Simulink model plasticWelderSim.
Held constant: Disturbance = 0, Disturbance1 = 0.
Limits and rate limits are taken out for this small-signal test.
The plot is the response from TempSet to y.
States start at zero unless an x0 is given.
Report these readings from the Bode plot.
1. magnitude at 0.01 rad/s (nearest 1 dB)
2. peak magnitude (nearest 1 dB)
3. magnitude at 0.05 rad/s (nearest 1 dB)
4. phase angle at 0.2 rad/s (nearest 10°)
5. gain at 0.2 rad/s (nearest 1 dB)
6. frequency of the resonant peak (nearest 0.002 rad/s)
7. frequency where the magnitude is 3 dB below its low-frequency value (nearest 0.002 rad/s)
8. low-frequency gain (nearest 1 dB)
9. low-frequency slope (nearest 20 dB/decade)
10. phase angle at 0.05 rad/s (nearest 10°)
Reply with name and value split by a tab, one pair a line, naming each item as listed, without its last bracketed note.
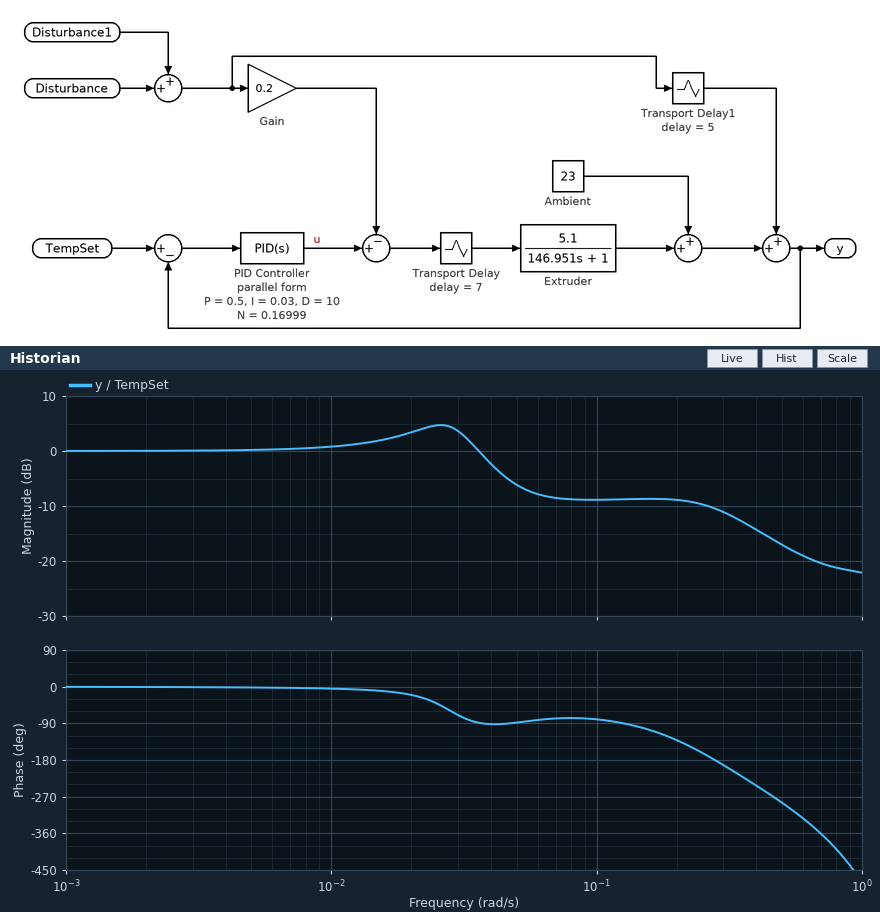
magnitude at 0.01 rad/s	1 dB
peak magnitude	5 dB
magnitude at 0.05 rad/s	-6 dB
phase angle at 0.2 rad/s	-130°
gain at 0.2 rad/s	-9 dB
frequency of the resonant peak	0.026 rad/s
frequency where the magnitude is 3 dB below its low-frequency value	0.042 rad/s
low-frequency gain	0 dB
low-frequency slope	0 dB/decade
phase angle at 0.05 rad/s	-90°
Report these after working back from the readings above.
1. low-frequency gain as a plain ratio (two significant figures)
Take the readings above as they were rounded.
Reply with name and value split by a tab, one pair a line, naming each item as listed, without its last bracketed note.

low-frequency gain as a plain ratio	1.0
